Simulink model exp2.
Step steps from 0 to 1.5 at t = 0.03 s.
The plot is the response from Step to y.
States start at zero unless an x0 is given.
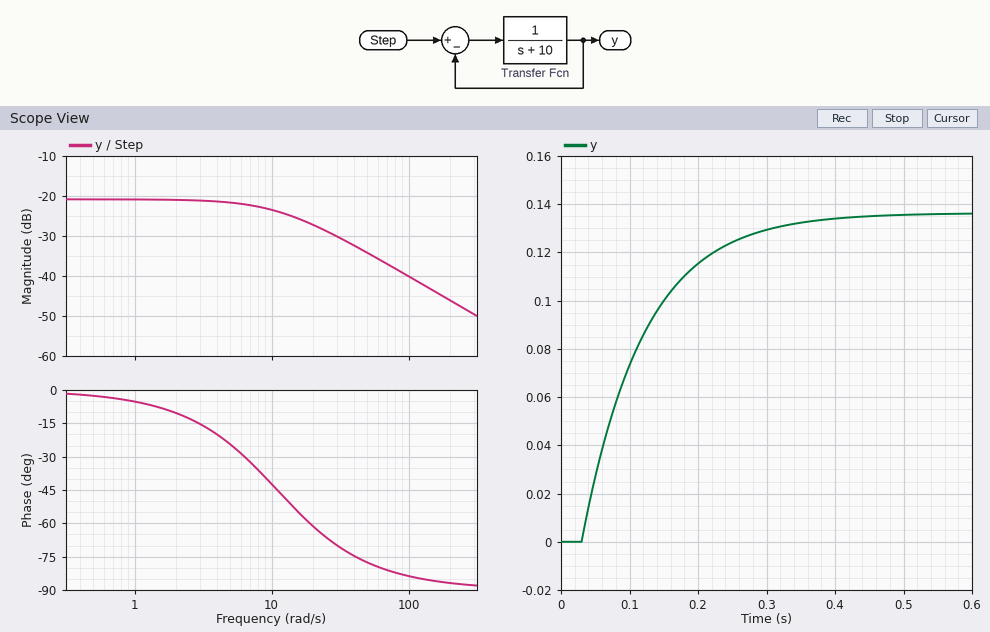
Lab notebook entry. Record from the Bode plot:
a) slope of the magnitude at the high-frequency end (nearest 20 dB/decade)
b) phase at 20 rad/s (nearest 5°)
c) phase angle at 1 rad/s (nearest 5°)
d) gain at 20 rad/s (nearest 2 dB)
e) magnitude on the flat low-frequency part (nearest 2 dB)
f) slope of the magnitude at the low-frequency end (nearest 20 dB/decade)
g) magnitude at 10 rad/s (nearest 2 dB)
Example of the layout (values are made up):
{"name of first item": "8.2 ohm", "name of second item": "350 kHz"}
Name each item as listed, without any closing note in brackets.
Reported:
{"slope of the magnitude at the high-frequency end": "-20 dB/decade", "phase at 20 rad/s": "-60°", "phase angle at 1 rad/s": "-5°", "gain at 20 rad/s": "-28 dB", "magnitude on the flat low-frequency part": "-20 dB", "slope of the magnitude at the low-frequency end": "0 dB/decade", "magnitude at 10 rad/s": "-24 dB"}
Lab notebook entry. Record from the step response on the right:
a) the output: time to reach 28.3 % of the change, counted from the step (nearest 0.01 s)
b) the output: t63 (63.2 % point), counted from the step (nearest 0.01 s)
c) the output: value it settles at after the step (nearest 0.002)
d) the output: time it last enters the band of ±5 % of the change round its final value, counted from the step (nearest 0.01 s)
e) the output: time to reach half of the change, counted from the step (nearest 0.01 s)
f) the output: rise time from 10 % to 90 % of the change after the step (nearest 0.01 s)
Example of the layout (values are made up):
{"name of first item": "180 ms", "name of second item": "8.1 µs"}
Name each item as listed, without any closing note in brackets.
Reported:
{"the output: time to reach 28.3 % of the change, counted from the step": "0.03 s", "the output: t63 (63.2 % point), counted from the step": "0.09 s", "the output: value it settles at after the step": "0.136", "the output: time it last enters the band of ±5 % of the change round its final value, counted from the step": "0.27 s", "the output: time to reach half of the change, counted from the step": "0.06 s", "the output: rise time from 10 % to 90 % of the change after the step": "0.20 s"}
